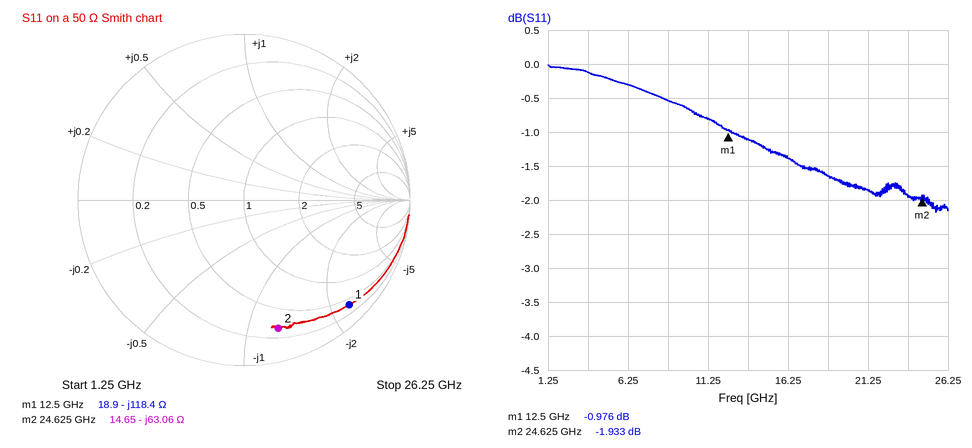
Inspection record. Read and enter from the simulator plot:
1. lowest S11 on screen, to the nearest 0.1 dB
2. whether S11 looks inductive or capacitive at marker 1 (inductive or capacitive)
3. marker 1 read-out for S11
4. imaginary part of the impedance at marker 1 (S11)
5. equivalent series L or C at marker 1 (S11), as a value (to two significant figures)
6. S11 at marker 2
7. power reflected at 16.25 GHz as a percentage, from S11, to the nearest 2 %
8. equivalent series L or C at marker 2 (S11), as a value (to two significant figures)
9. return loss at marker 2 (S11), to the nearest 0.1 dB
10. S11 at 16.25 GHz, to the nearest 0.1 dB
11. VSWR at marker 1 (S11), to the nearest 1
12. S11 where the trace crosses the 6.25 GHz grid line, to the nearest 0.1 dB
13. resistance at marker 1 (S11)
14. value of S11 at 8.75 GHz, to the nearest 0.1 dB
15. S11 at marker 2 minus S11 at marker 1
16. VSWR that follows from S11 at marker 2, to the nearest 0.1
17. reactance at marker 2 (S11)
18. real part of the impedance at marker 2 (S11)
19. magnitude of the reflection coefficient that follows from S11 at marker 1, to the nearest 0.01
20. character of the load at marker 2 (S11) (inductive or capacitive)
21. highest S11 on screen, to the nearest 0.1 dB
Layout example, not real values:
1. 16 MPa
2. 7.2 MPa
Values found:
1. -2.2 dB
2. capacitive
3. -0.976 dB
4. -118.4 Ω
5. 110 fF
6. -1.933 dB
7. 72 %
8. 100 fF
9. 1.9 dB
10. -1.4 dB
11. 18
12. -0.3 dB
13. 18.9 Ω
14. -0.5 dB
15. -0.957 dB
16. 9.0
17. -63.06 Ω
18. 14.65 Ω
19. 0.89
20. capacitive
21. 0.0 dB
